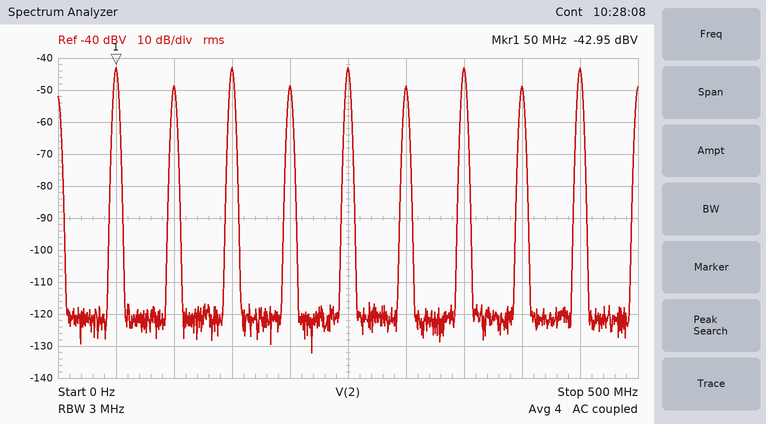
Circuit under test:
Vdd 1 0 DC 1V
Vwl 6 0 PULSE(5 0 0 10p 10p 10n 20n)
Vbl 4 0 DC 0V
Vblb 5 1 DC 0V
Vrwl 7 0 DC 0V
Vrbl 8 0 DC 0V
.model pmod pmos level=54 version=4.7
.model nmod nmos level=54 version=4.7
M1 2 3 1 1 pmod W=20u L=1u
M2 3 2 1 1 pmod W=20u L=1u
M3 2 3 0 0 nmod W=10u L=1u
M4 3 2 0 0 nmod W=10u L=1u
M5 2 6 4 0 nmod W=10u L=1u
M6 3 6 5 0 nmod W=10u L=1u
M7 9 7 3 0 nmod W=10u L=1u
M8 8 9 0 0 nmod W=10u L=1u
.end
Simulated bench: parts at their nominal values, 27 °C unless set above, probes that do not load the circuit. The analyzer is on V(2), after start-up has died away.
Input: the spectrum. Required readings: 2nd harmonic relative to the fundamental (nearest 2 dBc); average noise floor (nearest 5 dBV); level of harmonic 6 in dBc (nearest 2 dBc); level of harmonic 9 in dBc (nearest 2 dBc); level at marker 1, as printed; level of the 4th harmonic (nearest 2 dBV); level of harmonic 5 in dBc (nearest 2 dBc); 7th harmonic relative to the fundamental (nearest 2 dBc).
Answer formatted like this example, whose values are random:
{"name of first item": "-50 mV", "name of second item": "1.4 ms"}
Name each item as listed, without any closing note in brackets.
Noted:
{"2nd harmonic relative to the fundamental": "-6 dBc", "average noise floor": "-120 dBV", "level of harmonic 6 in dBc": "-6 dBc", "level of harmonic 9 in dBc": "0 dBc", "level at marker 1, as printed": "-42.95 dBV", "level of the 4th harmonic": "-48 dBV", "level of harmonic 5 in dBc": "0 dBc", "7th harmonic relative to the fundamental": "0 dBc"}
